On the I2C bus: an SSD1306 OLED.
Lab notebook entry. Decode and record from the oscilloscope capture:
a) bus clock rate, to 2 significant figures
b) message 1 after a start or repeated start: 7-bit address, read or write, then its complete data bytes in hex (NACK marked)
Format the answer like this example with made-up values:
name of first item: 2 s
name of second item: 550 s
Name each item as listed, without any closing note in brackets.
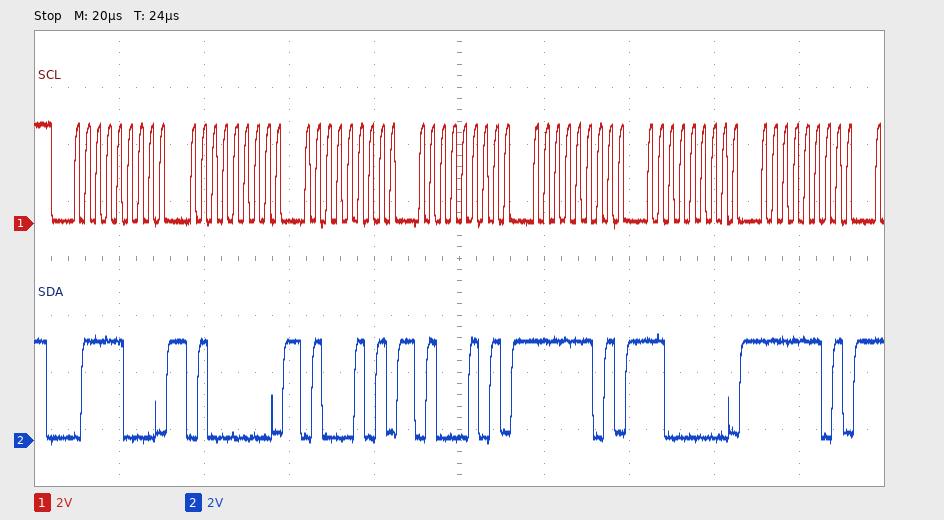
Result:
bus clock rate, to 2 significant figures: 400 kHz
message 1 after a start or repeated start: 7-bit address, read or write, then its complete data bytes in hex: 0x3C write: 40 45 45 FD C0 FD
